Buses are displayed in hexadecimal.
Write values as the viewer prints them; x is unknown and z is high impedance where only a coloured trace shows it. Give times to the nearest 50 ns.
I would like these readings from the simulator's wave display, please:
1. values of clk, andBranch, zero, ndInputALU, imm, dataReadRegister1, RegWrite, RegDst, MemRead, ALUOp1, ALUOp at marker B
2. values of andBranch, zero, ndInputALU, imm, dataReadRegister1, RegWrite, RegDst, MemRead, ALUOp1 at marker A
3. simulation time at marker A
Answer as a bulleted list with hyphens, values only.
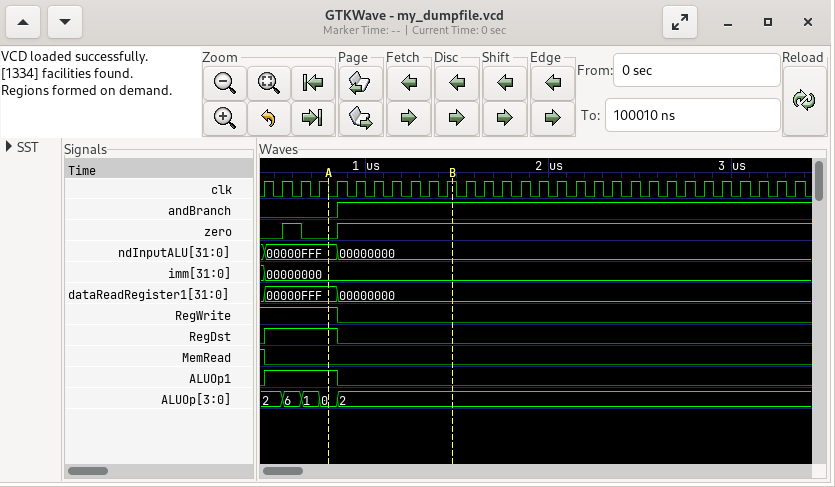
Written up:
- clk=1, andBranch=1, zero=1, ndInputALU=00000000, imm=00000000, dataReadRegister1=00000000, RegWrite=0, RegDst=0, MemRead=0, ALUOp1=0, ALUOp=2
- andBranch=0, zero=0, ndInputALU=00000FFF, imm=00000000, dataReadRegister1=00000FFF, RegWrite=1, RegDst=1, MemRead=0, ALUOp1=1
- 800 ns
